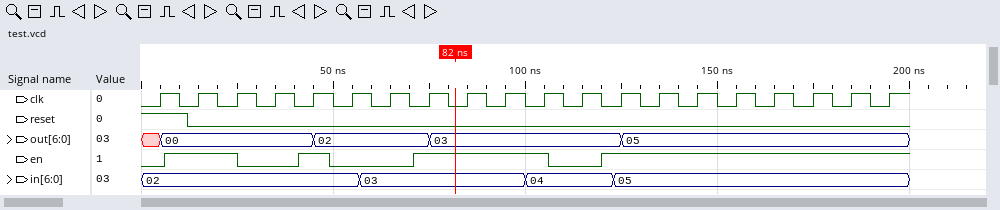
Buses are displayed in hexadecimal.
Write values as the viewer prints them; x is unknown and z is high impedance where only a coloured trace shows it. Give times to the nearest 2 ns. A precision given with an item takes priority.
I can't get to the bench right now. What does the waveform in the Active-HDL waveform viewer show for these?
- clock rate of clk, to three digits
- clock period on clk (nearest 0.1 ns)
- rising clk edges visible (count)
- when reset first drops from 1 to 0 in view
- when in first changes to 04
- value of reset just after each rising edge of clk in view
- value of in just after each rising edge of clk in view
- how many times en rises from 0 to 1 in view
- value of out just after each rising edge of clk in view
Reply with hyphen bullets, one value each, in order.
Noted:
- 100 MHz
- 10 ns
- 20
- 12 ns
- 100 ns
- 1 0 0 0 0 0 0 0 0 0 0 0 0 0 0 0 0 0 0 0
- 02, 02, 02, 02, 02, 02, 03, 03, 03, 03, 04, 04, 05, 05, 05, 05, 05, 05, 05, 05
- 4
- 00, 00, 00, 00, 02, 02, 02, 03, 03, 03, 03, 03, 05, 05, 05, 05, 05, 05, 05, 05
